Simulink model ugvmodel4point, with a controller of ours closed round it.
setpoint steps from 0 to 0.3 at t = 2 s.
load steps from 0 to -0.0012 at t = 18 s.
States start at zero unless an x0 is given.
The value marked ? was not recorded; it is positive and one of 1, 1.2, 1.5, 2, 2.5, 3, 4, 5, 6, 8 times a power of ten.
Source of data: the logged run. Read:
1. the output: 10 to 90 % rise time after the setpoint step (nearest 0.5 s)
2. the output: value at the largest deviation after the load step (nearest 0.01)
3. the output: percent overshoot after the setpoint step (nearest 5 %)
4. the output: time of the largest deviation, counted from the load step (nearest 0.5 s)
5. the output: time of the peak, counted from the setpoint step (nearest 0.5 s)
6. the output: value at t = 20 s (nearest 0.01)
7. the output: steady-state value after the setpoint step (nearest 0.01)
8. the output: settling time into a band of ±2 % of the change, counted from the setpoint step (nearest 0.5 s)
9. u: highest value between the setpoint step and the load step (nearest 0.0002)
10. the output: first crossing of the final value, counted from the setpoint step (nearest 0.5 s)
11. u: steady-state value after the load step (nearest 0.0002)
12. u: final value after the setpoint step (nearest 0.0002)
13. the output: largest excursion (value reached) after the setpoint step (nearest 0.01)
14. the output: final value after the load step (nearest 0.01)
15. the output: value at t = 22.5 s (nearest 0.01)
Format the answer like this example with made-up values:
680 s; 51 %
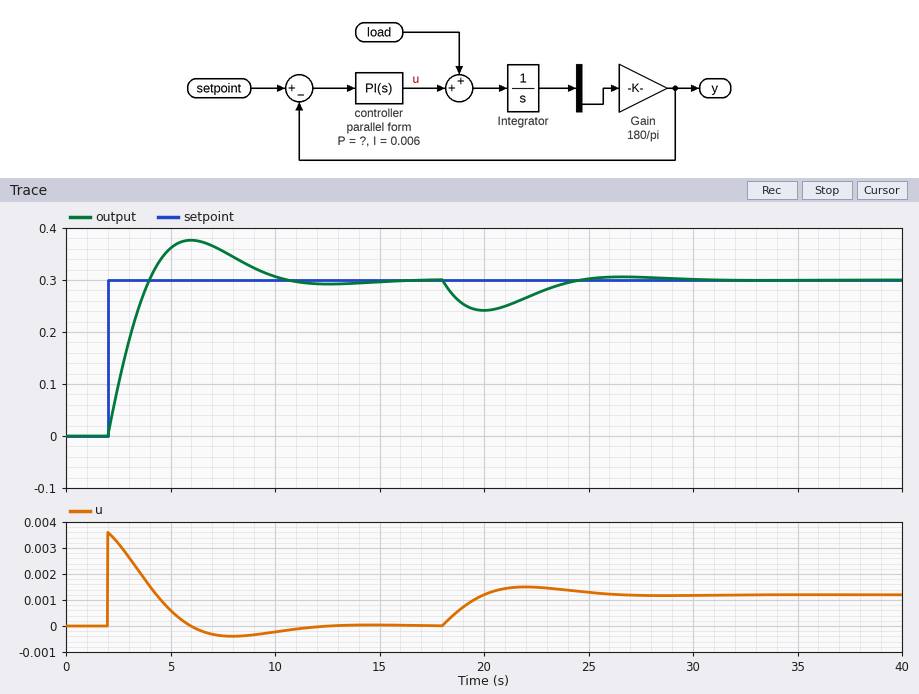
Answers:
1.5 s; 0.24; 25 %; 2.0 s; 4.0 s; 0.24; 0.30; 12.0 s; 0.0036; 2.0 s; 0.0012; 0.0000; 0.38; 0.30; 0.27
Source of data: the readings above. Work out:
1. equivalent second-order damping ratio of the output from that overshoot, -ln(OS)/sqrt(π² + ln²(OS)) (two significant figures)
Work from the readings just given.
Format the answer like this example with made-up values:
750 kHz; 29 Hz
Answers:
0.40
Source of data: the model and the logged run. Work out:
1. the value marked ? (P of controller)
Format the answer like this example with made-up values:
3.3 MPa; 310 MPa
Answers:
0.012
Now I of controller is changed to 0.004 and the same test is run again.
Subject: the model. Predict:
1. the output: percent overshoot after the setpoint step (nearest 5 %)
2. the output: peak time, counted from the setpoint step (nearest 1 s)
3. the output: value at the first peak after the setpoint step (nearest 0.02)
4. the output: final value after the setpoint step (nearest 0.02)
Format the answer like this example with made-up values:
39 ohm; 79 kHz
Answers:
20 %; 5 s; 0.36; 0.30
